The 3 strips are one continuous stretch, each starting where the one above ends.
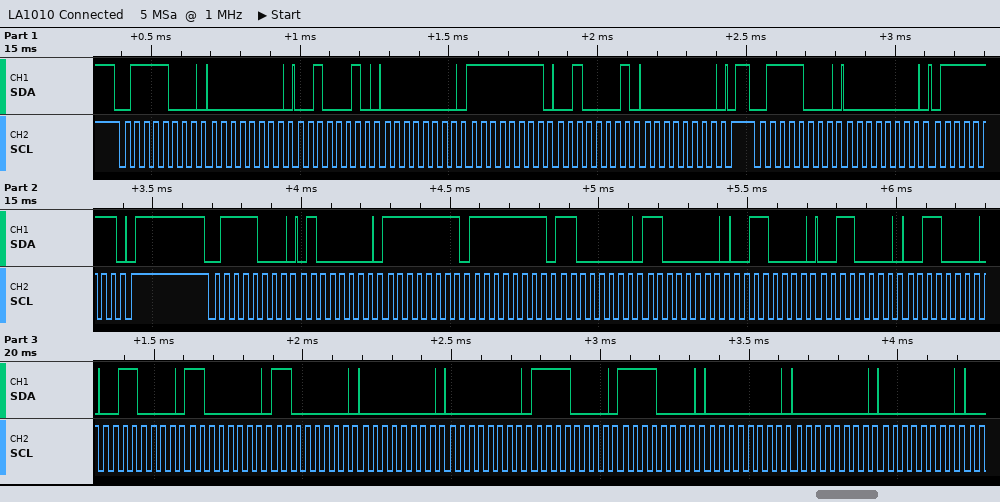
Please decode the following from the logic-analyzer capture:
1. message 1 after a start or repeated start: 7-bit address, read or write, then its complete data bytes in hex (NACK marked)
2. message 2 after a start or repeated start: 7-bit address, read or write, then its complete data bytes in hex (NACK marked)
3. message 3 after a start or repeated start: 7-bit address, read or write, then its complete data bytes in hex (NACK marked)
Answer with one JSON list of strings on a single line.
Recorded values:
["0x3C write: 00 22 00 FF 21 00", "0x3C write: 00 7F", "0x3C write: 40 FF FF C0 C0 30 30 30 30 C0 C0 00 00 F0 F0 00 00 00"]
